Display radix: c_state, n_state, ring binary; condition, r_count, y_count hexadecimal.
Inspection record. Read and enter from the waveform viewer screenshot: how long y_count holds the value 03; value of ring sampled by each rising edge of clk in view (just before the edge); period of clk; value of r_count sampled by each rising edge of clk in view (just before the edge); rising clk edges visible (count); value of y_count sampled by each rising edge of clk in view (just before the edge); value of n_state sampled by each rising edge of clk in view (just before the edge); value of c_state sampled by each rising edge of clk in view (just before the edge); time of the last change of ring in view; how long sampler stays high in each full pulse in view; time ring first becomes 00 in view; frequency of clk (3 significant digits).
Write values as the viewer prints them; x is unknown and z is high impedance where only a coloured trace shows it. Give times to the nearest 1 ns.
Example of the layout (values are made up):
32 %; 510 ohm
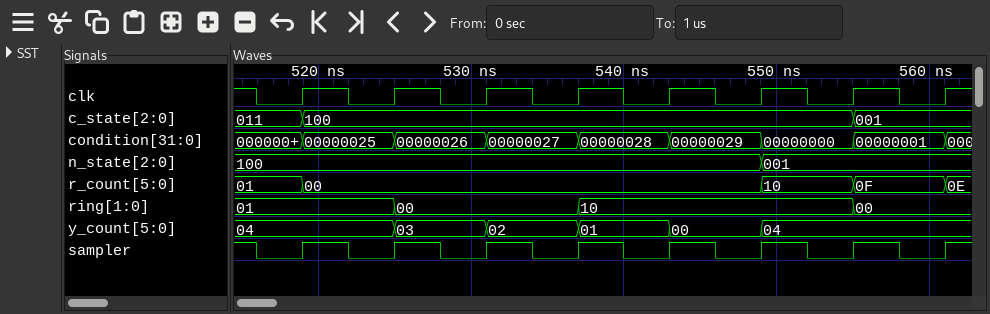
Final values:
6 ns; 01, 01, 00, 00, 10, 10, 10, 00; 6 ns; 01, 00, 00, 00, 00, 00, 10, 0F; 8; 04, 04, 03, 02, 01, 00, 04, 04; 100, 100, 100, 100, 100, 100, 001, 001; 011, 100, 100, 100, 100, 100, 100, 001; 555 ns; 3 ns, 3 ns, 3 ns, 3 ns, 3 ns, 3 ns, 3 ns; 525 ns; 167 MHz
